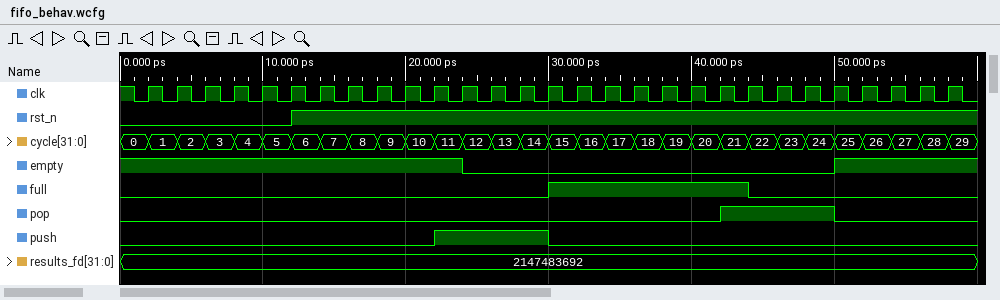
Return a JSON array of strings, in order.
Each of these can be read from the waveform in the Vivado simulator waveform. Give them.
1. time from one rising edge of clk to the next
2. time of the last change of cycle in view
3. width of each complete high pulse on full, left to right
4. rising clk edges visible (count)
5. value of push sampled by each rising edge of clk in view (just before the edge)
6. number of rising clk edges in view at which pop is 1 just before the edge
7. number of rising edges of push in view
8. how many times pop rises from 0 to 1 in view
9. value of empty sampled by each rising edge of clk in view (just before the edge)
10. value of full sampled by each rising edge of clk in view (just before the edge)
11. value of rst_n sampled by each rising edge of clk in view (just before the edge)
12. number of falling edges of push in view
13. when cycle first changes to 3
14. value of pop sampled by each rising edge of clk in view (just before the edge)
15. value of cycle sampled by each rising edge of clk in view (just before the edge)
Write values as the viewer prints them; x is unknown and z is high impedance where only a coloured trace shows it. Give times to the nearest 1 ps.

["2 ps", "58 ps", "14 ps", "29", "0 0 0 0 0 0 0 0 0 0 0 1 1 1 1 0 0 0 0 0 0 0 0 0 0 0 0 0 0", "4", "1", "1", "1 1 1 1 1 1 1 1 1 1 1 1 0 0 0 0 0 0 0 0 0 0 0 0 0 1 1 1 1", "0 0 0 0 0 0 0 0 0 0 0 0 0 0 0 1 1 1 1 1 1 1 0 0 0 0 0 0 0", "0 0 0 0 0 0 1 1 1 1 1 1 1 1 1 1 1 1 1 1 1 1 1 1 1 1 1 1 1", "1", "6 ps", "0 0 0 0 0 0 0 0 0 0 0 0 0 0 0 0 0 0 0 0 0 1 1 1 1 0 0 0 0", "0, 1, 2, 3, 4, 5, 6, 7, 8, 9, 10, 11, 12, 13, 14, 15, 16, 17, 18, 19, 20, 21, 22, 23, 24, 25, 26, 27, 28"]
